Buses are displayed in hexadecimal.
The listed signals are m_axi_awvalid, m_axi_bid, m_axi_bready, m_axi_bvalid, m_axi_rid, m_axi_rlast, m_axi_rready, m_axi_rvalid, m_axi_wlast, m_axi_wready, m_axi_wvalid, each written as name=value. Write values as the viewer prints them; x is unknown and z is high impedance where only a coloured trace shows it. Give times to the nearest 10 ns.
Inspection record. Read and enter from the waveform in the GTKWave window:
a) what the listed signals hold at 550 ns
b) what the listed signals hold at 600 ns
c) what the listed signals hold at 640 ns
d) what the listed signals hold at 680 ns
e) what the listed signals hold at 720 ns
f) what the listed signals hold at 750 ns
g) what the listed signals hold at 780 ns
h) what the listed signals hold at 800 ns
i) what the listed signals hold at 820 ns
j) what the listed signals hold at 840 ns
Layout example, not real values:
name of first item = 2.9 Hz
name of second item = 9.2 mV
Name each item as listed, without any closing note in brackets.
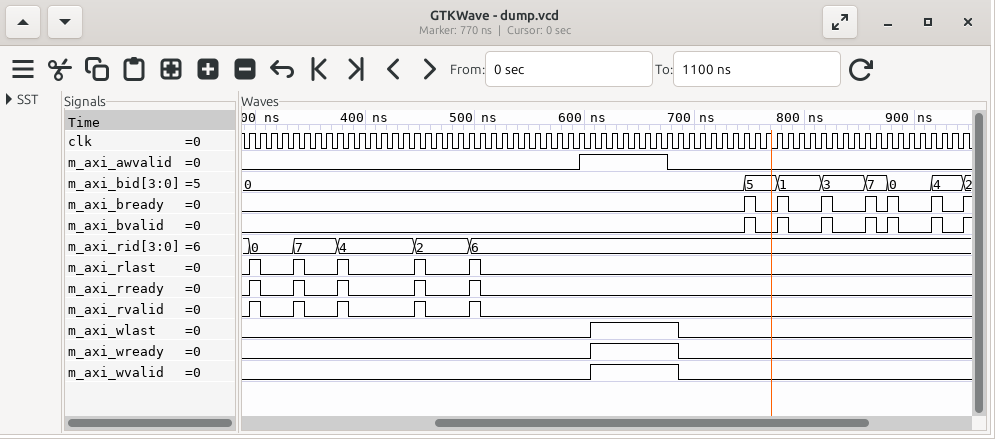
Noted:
what the listed signals hold at 550 ns = m_axi_awvalid=0, m_axi_bid=0, m_axi_bready=0, m_axi_bvalid=0, m_axi_rid=6, m_axi_rlast=0, m_axi_rready=0, m_axi_rvalid=0, m_axi_wlast=0, m_axi_wready=0, m_axi_wvalid=0
what the listed signals hold at 600 ns = m_axi_awvalid=1, m_axi_bid=0, m_axi_bready=0, m_axi_bvalid=0, m_axi_rid=6, m_axi_rlast=0, m_axi_rready=0, m_axi_rvalid=0, m_axi_wlast=0, m_axi_wready=0, m_axi_wvalid=0
what the listed signals hold at 640 ns = m_axi_awvalid=1, m_axi_bid=0, m_axi_bready=0, m_axi_bvalid=0, m_axi_rid=6, m_axi_rlast=0, m_axi_rready=0, m_axi_rvalid=0, m_axi_wlast=1, m_axi_wready=1, m_axi_wvalid=1
what the listed signals hold at 680 ns = m_axi_awvalid=0, m_axi_bid=0, m_axi_bready=0, m_axi_bvalid=0, m_axi_rid=6, m_axi_rlast=0, m_axi_rready=0, m_axi_rvalid=0, m_axi_wlast=1, m_axi_wready=1, m_axi_wvalid=1
what the listed signals hold at 720 ns = m_axi_awvalid=0, m_axi_bid=0, m_axi_bready=0, m_axi_bvalid=0, m_axi_rid=6, m_axi_rlast=0, m_axi_rready=0, m_axi_rvalid=0, m_axi_wlast=0, m_axi_wready=0, m_axi_wvalid=0
what the listed signals hold at 750 ns = m_axi_awvalid=0, m_axi_bid=5, m_axi_bready=1, m_axi_bvalid=1, m_axi_rid=6, m_axi_rlast=0, m_axi_rready=0, m_axi_rvalid=0, m_axi_wlast=0, m_axi_wready=0, m_axi_wvalid=0
what the listed signals hold at 780 ns = m_axi_awvalid=0, m_axi_bid=1, m_axi_bready=1, m_axi_bvalid=1, m_axi_rid=6, m_axi_rlast=0, m_axi_rready=0, m_axi_rvalid=0, m_axi_wlast=0, m_axi_wready=0, m_axi_wvalid=0
what the listed signals hold at 800 ns = m_axi_awvalid=0, m_axi_bid=1, m_axi_bready=0, m_axi_bvalid=0, m_axi_rid=6, m_axi_rlast=0, m_axi_rready=0, m_axi_rvalid=0, m_axi_wlast=0, m_axi_wready=0, m_axi_wvalid=0
what the listed signals hold at 820 ns = m_axi_awvalid=0, m_axi_bid=3, m_axi_bready=1, m_axi_bvalid=1, m_axi_rid=6, m_axi_rlast=0, m_axi_rready=0, m_axi_rvalid=0, m_axi_wlast=0, m_axi_wready=0, m_axi_wvalid=0
what the listed signals hold at 840 ns = m_axi_awvalid=0, m_axi_bid=3, m_axi_bready=0, m_axi_bvalid=0, m_axi_rid=6, m_axi_rlast=0, m_axi_rready=0, m_axi_rvalid=0, m_axi_wlast=0, m_axi_wready=0, m_axi_wvalid=0
